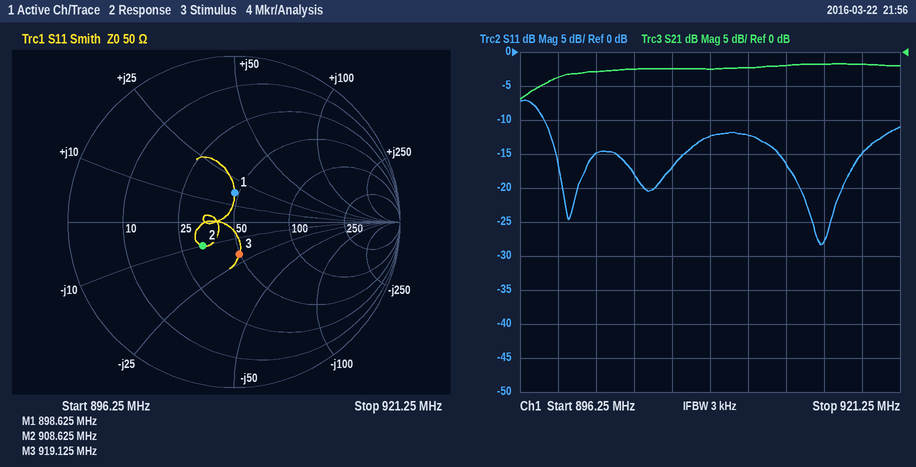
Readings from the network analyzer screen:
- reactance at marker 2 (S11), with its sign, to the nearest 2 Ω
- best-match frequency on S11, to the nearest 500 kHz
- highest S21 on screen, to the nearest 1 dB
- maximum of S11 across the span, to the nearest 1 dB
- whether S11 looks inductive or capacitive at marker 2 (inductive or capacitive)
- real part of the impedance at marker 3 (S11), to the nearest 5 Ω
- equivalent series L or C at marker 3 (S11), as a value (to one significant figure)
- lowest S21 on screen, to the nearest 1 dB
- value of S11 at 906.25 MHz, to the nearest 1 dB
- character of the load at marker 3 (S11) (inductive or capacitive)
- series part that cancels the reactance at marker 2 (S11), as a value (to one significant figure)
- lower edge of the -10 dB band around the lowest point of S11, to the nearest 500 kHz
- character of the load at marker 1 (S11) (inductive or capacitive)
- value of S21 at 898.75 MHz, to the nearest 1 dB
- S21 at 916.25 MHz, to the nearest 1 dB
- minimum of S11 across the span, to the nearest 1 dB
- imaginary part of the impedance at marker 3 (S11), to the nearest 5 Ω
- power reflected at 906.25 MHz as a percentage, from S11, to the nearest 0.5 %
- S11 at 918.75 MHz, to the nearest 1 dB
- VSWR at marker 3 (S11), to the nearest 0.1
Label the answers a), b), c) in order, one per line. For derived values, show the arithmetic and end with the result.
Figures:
a) -10 Ω
b) 916.0 MHz
c) -2 dB
d) -7 dB
e) capacitive
f) 50 Ω
g) C = 1/(2π × 919.125 MHz × 20 Ω) ≈ 9 pF
h) -7 dB
i) -17 dB
j) capacitive
k) L = 10 Ω/(2π × 908.625 MHz) ≈ 2 nH
l) 898.0 MHz
m) inductive
n) -4 dB
o) -2 dB
p) -28 dB
q) -20 Ω
r) 10^(-17/10) ≈ 2.0 %
s) -15 dB
t) 1.5
